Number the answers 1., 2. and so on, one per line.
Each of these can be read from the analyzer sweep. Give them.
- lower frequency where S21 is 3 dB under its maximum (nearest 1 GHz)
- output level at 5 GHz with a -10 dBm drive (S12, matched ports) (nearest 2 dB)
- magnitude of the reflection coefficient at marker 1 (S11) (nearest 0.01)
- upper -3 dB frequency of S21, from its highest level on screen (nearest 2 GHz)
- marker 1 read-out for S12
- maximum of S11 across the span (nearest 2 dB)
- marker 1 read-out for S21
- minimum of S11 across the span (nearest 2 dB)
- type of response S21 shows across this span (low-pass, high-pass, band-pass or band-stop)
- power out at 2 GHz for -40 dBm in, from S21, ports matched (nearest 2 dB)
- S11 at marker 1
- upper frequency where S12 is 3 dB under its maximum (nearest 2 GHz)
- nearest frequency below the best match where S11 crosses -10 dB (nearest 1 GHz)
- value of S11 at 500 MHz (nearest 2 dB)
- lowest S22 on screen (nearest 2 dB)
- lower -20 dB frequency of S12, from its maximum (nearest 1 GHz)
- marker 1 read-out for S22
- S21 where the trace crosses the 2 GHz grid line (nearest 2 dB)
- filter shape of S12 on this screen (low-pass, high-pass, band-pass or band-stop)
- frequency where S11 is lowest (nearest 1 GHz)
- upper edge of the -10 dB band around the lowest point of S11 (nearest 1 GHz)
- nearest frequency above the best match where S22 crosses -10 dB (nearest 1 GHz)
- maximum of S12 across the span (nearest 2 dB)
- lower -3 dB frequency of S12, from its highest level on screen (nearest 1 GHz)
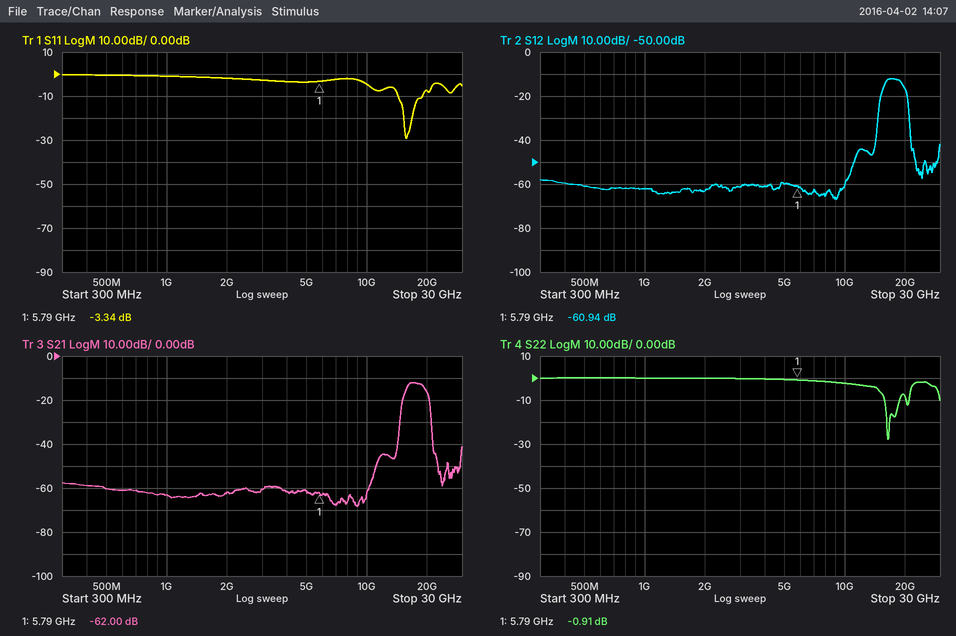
1. 16 GHz
2. -70 dBm
3. 0.68
4. 20 GHz
5. -60.94 dB
6. 0 dB
7. -62.00 dB
8. -30 dB
9. band-pass
10. -102 dBm
11. -3.34 dB
12. 20 GHz
13. 14 GHz
14. 0 dB
15. -28 dB
16. 15 GHz
17. -0.91 dB
18. -62 dB
19. band-pass
20. 16 GHz
21. 19 GHz
22. 19 GHz
23. -12 dB
24. 16 GHz
